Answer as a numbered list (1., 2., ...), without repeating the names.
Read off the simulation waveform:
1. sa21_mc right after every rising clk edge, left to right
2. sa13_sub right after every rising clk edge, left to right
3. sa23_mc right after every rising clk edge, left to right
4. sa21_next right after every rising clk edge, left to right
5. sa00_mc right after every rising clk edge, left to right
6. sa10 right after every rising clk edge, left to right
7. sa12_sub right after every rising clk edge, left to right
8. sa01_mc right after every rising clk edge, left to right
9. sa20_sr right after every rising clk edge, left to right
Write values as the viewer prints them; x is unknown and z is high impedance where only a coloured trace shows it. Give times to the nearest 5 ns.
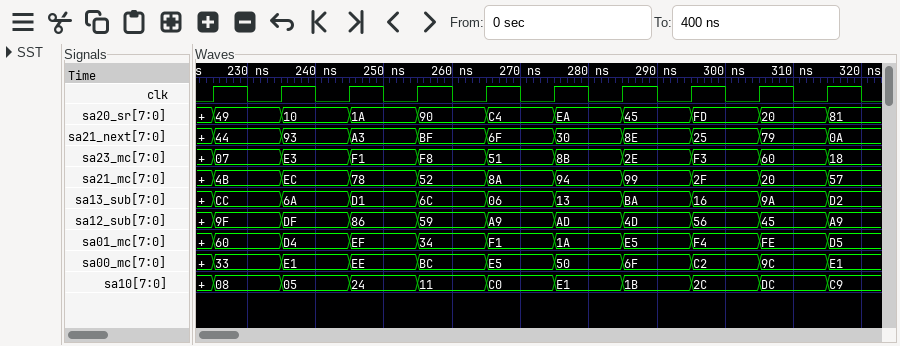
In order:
1. 4B, EC, 78, 52, 8A, 94, 99, 2F, 20, 57
2. CC, 6A, D1, 6C, 06, 13, BA, 16, 9A, D2
3. 07, E3, F1, F8, 51, 8B, 2E, F3, 60, 18
4. 44, 93, A3, BF, 6F, 30, 8E, 25, 79, 0A
5. 33, E1, EE, BC, E5, 50, 6F, C2, 9C, E1
6. 08, 05, 24, 11, C0, E1, 1B, 2C, DC, C9
7. 9F, DF, 86, 59, A9, AD, 4D, 56, 45, A9
8. 60, D4, EF, 34, F1, 1A, E5, F4, FE, D5
9. 49, 10, 1A, 90, C4, EA, 45, FD, 20, 81
